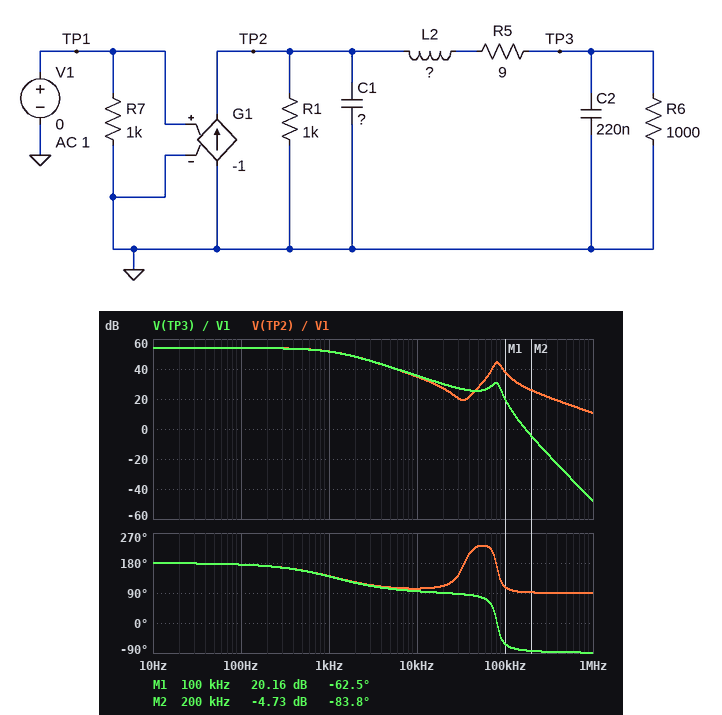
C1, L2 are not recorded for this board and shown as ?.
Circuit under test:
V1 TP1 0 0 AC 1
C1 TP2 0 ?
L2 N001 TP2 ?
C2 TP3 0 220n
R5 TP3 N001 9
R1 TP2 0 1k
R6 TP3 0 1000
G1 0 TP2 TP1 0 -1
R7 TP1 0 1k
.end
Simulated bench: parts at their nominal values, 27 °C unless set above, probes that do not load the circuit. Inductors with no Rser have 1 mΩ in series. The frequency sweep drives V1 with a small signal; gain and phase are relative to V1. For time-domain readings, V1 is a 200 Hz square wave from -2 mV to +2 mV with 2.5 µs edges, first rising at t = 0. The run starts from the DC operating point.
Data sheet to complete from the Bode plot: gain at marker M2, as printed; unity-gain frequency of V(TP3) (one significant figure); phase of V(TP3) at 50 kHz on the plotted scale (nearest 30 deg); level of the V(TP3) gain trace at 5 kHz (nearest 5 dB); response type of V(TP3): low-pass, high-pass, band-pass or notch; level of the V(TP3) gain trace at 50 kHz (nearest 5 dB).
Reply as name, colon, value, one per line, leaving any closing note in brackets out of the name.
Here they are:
gain at marker M2, as printed: -4.73 dB
unity-gain frequency of V(TP3): 200 kHz
phase of V(TP3) at 50 kHz on the plotted scale: 90 deg
level of the V(TP3) gain trace at 5 kHz: 40 dB
response type of V(TP3): low-pass, high-pass, band-pass or notch: low-pass
level of the V(TP3) gain trace at 50 kHz: 25 dB
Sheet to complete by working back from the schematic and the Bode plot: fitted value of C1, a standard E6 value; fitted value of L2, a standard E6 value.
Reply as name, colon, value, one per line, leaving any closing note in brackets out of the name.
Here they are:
fitted value of C1, a standard E6 value: 47 nF
fitted value of L2, a standard E6 value: 100 µH
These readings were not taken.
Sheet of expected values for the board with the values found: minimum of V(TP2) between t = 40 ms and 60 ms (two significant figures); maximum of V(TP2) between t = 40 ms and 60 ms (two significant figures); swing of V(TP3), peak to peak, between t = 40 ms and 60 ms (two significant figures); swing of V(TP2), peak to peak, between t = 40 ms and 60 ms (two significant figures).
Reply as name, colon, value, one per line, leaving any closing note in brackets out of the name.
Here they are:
minimum of V(TP2) between t = 40 ms and 60 ms: -1.0 V
maximum of V(TP2) between t = 40 ms and 60 ms: 1.0 V
swing of V(TP3), peak to peak, between t = 40 ms and 60 ms: 2.0 V
swing of V(TP2), peak to peak, between t = 40 ms and 60 ms: 2.0 V
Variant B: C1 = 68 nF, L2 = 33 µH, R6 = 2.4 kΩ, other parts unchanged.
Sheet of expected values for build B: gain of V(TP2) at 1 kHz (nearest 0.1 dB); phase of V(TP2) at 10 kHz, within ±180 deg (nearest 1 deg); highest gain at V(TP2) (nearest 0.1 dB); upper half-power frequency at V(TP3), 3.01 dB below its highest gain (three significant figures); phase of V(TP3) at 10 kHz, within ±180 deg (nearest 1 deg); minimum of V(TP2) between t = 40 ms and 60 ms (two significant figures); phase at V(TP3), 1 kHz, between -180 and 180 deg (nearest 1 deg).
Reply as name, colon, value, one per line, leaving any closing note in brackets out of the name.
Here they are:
gain of V(TP2) at 1 kHz: 52.8 dB
phase of V(TP2) at 10 kHz, within ±180 deg: 100 deg
highest gain at V(TP2): 57.0 dB
upper half-power frequency at V(TP3), 3.01 dB below its highest gain: 781 Hz
phase of V(TP3) at 10 kHz, within ±180 deg: 93 deg
minimum of V(TP2) between t = 40 ms and 60 ms: -1.4 V
phase at V(TP3), 1 kHz, between -180 and 180 deg: 128 deg
